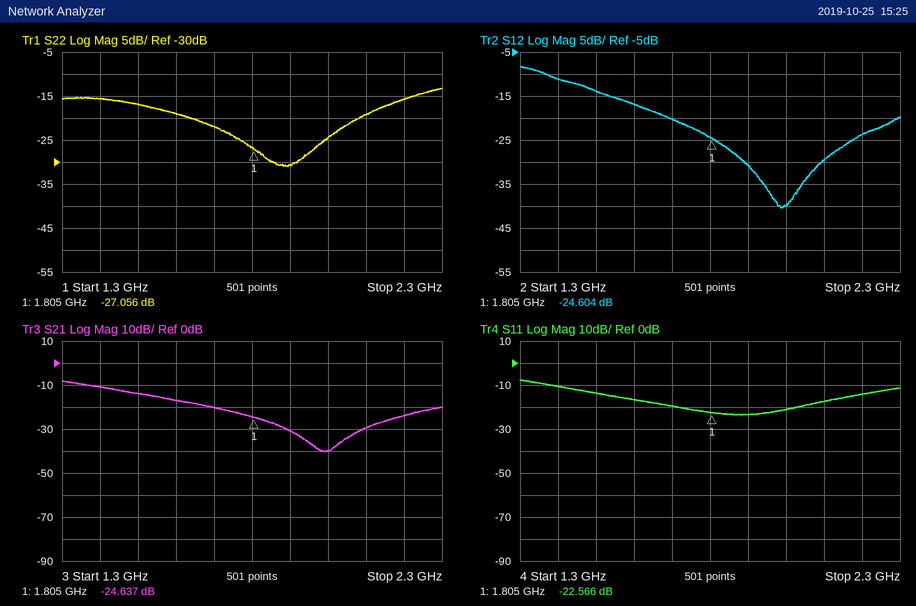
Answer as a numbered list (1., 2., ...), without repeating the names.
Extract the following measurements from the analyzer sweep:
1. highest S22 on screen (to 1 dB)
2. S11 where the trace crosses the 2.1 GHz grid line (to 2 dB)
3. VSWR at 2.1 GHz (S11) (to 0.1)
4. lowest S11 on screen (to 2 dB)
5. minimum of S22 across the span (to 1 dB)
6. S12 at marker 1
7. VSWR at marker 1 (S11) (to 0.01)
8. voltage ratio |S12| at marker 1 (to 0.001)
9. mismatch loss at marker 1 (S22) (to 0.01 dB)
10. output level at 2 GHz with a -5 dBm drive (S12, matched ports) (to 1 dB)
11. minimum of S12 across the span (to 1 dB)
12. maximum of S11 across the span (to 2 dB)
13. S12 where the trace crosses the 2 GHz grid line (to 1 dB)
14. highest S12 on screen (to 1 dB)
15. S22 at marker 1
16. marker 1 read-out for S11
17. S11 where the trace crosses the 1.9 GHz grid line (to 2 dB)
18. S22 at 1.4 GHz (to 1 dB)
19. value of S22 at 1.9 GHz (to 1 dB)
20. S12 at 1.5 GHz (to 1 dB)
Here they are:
1. -13 dB
2. -18 dB
3. 1.3
4. -24 dB
5. -31 dB
6. -24.604 dB
7. 1.16
8. 0.059
9. 0.01 dB
10. -45 dBm
11. -40 dB
12. -8 dB
13. -40 dB
14. -8 dB
15. -27.056 dB
16. -22.566 dB
17. -24 dB
18. -16 dB
19. -31 dB
20. -14 dB
